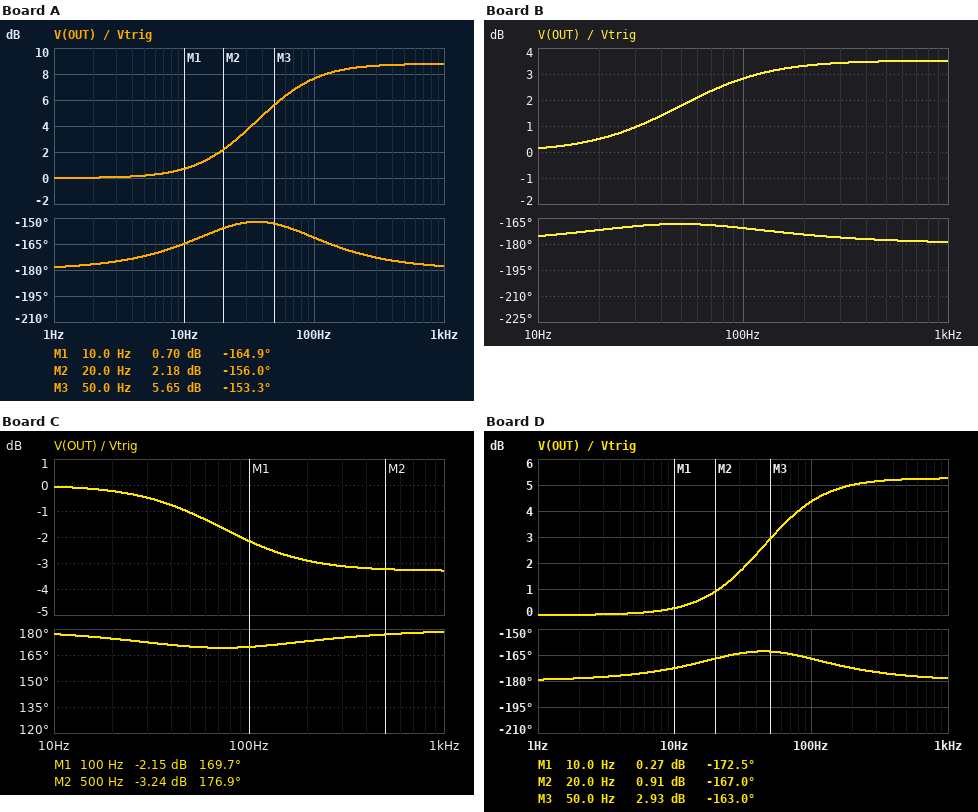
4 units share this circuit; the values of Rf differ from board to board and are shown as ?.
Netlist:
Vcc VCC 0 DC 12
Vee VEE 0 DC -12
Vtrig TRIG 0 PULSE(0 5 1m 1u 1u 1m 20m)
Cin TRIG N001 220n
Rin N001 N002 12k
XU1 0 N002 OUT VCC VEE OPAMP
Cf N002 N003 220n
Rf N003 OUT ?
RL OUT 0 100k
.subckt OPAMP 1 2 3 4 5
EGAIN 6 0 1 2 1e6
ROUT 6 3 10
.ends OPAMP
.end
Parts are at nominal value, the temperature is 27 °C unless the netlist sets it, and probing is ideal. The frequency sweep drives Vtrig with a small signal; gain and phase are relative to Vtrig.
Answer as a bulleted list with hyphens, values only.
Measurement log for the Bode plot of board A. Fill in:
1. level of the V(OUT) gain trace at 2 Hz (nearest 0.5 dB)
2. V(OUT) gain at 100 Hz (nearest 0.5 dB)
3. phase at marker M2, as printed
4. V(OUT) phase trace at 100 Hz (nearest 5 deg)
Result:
- 0 dB
- 7.5 dB
- -156.0 deg
- -160 deg
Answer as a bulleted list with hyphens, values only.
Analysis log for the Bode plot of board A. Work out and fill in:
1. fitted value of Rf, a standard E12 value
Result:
- 33 kΩ
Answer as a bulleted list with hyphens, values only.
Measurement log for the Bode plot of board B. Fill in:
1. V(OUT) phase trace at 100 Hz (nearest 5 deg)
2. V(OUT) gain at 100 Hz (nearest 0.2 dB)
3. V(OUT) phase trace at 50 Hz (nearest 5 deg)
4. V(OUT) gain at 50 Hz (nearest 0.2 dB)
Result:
- -170 deg
- 2.8 dB
- -170 deg
- 1.8 dB
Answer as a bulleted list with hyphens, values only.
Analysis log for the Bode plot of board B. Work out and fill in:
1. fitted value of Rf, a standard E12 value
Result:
- 18 kΩ
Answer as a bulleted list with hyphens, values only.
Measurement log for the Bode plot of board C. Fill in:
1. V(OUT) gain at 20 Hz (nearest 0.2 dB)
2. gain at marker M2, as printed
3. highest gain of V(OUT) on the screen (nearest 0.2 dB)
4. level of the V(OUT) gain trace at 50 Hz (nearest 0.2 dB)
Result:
- -0.2 dB
- -3.24 dB
- 0 dB
- -1.0 dB
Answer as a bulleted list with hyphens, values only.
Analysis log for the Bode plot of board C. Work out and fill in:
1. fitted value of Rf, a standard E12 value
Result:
- 8.2 kΩ
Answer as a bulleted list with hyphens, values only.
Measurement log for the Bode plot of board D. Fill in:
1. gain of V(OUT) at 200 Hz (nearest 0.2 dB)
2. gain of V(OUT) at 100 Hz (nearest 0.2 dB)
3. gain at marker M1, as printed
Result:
- 5.0 dB
- 4.4 dB
- 0.27 dB
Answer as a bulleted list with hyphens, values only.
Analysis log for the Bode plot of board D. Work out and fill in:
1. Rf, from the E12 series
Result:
- 22 kΩ
